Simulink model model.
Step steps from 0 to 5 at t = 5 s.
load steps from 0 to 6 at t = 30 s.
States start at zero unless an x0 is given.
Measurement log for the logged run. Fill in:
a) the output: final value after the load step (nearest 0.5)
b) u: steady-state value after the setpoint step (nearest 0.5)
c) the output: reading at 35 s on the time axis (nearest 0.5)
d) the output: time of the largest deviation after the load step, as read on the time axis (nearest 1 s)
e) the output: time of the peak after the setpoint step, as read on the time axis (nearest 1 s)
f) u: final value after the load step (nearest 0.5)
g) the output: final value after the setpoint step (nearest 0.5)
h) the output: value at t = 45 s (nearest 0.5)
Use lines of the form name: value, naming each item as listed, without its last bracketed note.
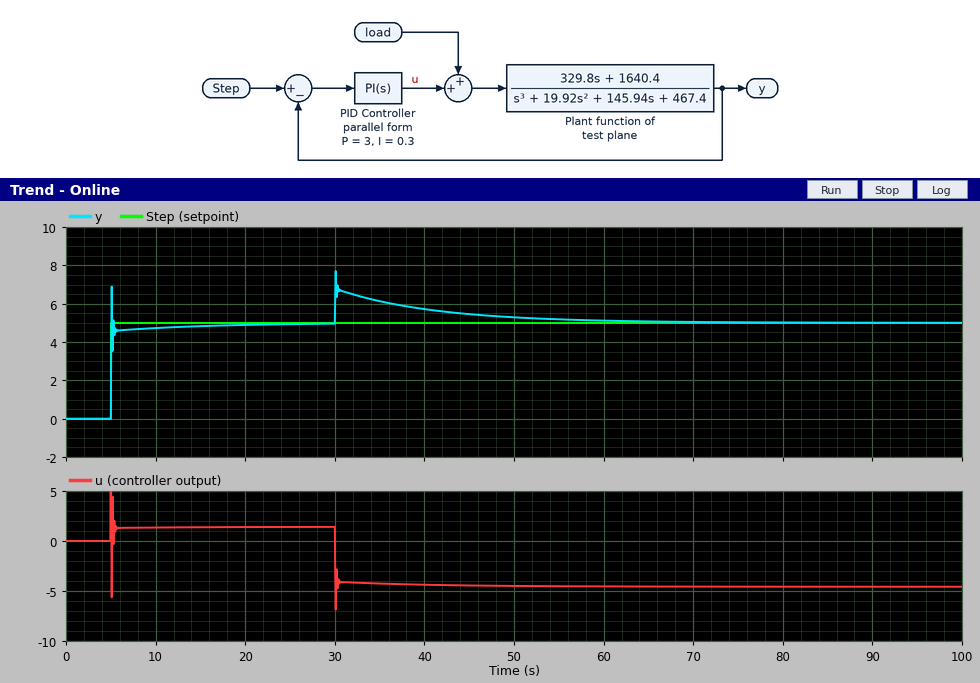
the output: final value after the load step: 5.0
u: steady-state value after the setpoint step: 1.5
the output: reading at 35 s on the time axis: 6.0
the output: time of the largest deviation after the load step, as read on the time axis: 30 s
the output: time of the peak after the setpoint step, as read on the time axis: 5 s
u: final value after the load step: -4.5
the output: final value after the setpoint step: 5.0
the output: value at t = 45 s: 5.5
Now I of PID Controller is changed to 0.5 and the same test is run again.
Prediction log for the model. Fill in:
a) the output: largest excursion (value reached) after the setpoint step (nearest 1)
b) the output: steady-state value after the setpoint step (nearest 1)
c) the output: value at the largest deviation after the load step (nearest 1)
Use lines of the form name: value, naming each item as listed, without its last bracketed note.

the output: largest excursion (value reached) after the setpoint step: 7
the output: steady-state value after the setpoint step: 5
the output: value at the largest deviation after the load step: 8
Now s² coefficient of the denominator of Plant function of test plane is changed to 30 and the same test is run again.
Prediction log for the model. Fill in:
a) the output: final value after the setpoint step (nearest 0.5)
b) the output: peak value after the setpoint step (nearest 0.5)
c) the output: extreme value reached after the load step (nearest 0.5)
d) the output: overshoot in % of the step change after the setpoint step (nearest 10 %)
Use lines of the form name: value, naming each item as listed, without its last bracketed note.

the output: final value after the setpoint step: 5.0
the output: peak value after the setpoint step: 6.0
the output: extreme value reached after the load step: 7.5
the output: overshoot in % of the step change after the setpoint step: 20 %
